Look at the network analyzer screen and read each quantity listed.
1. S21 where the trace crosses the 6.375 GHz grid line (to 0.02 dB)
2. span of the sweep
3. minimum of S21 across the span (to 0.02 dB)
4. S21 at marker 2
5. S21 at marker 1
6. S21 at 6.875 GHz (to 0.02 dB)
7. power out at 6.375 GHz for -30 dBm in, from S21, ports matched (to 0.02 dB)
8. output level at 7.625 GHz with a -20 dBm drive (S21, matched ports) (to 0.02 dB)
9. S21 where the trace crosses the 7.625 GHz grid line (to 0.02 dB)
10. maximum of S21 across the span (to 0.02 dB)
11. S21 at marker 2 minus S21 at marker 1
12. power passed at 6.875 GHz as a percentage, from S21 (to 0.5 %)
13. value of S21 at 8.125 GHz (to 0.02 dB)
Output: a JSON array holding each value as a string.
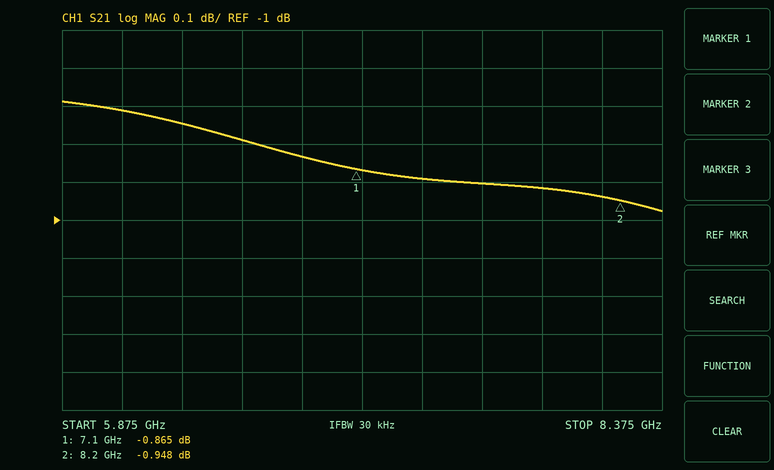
["-0.74 dB", "2.5 GHz", "-0.98 dB", "-0.948 dB", "-0.865 dB", "-0.84 dB", "-30.74 dBm", "-20.90 dBm", "-0.90 dB", "-0.68 dB", "-0.083 dB", "82.5 %", "-0.94 dB"]
